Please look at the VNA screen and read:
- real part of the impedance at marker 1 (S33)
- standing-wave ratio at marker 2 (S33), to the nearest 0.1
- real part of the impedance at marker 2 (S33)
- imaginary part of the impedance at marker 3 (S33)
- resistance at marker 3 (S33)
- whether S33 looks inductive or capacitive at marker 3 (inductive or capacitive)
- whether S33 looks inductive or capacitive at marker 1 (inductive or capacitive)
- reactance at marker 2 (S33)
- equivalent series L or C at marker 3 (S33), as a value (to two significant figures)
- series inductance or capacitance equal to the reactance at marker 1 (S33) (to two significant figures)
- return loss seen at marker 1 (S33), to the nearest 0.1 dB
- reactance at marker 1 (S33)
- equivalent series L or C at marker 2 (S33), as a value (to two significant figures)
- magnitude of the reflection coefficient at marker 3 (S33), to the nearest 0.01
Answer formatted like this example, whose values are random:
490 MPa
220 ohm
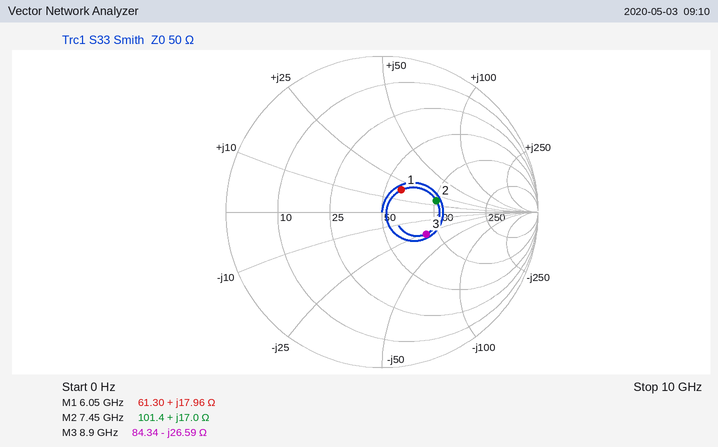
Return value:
61.30 Ω
2.1
101.4 Ω
-26.59 Ω
84.34 Ω
capacitive
inductive
+17.0 Ω
670 fF
470 pH
14.5 dB
+17.96 Ω
360 pH
0.32
